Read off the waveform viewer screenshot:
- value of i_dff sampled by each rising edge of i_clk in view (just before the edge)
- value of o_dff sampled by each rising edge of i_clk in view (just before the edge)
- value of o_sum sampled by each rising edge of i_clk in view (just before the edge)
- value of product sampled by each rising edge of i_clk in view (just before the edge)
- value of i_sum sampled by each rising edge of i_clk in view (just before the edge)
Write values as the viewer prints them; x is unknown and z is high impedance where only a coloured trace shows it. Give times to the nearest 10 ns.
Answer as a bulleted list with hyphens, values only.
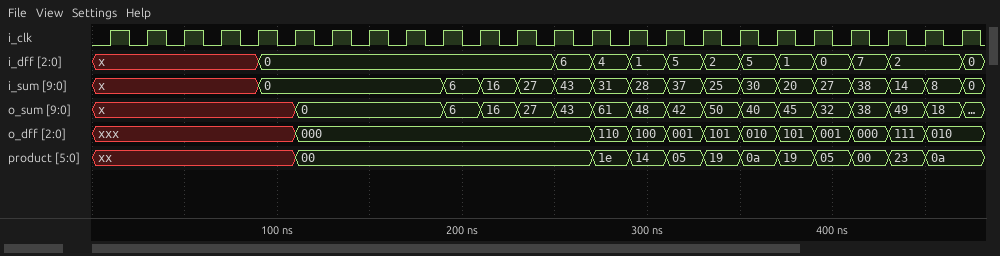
- x, x, x, x, x, 0, 0, 0, 0, 0, 0, 0, 0, 6, 4, 1, 5, 2, 5, 1, 0, 7, 2, 2
- xxx, xxx, xxx, xxx, xxx, xxx, 000, 000, 000, 000, 000, 000, 000, 000, 110, 100, 001, 101, 010, 101, 001, 000, 111, 010
- x, x, x, x, x, x, 0, 0, 0, 0, 6, 16, 27, 43, 61, 48, 42, 50, 40, 45, 32, 38, 49, 18
- xx, xx, xx, xx, xx, xx, 00, 00, 00, 00, 00, 00, 00, 00, 1e, 14, 05, 19, 0a, 19, 05, 00, 23, 0a
- x, x, x, x, x, 0, 0, 0, 0, 0, 6, 16, 27, 43, 31, 28, 37, 25, 30, 20, 27, 38, 14, 8
